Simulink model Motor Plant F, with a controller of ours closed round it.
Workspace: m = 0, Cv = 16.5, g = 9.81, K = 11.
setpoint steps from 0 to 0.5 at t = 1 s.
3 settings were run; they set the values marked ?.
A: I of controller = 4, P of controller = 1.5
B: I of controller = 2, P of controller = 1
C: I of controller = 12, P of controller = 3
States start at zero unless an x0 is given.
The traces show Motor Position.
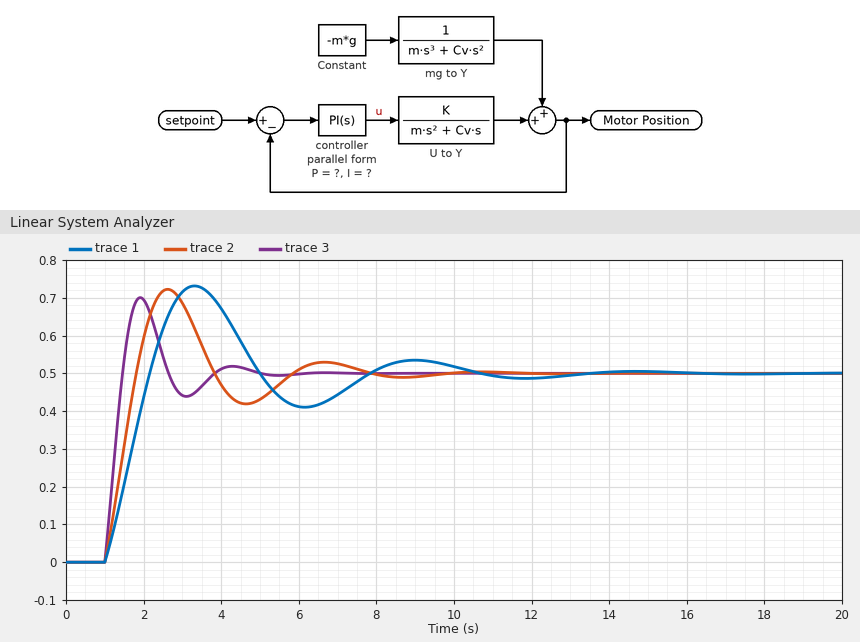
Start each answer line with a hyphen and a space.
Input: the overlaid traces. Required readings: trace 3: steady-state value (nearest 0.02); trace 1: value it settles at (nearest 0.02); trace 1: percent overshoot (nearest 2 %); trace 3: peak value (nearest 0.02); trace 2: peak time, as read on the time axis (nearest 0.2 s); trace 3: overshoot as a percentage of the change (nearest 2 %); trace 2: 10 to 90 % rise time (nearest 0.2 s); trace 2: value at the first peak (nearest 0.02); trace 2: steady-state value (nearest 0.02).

- 0.50
- 0.50
- 46 %
- 0.70
- 2.6 s
- 40 %
- 0.6 s
- 0.72
- 0.50
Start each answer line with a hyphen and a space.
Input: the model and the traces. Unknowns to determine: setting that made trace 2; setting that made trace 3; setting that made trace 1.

- A
- C
- B
